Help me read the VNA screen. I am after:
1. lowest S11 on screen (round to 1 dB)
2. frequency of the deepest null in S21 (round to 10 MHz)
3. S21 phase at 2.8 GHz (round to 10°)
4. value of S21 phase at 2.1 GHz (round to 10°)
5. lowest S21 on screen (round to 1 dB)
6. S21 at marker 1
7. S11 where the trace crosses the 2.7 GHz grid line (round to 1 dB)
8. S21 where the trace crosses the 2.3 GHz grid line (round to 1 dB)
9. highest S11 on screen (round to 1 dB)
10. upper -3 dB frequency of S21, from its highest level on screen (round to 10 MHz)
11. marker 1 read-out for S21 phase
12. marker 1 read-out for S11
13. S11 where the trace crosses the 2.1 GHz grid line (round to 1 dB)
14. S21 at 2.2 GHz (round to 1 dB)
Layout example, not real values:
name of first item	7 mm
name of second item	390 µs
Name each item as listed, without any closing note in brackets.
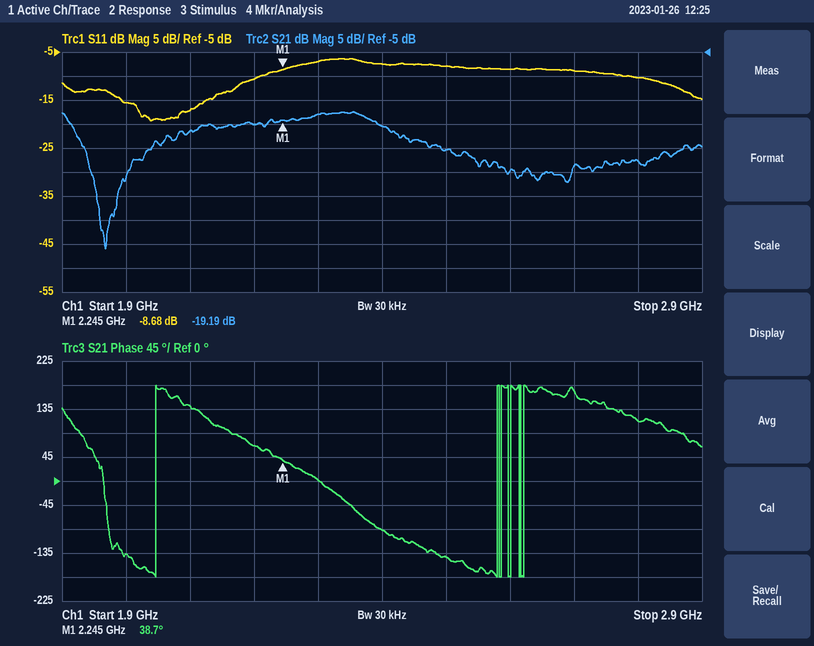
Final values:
lowest S11 on screen	-19 dB
frequency of the deepest null in S21	1.97 GHz
S21 phase at 2.8 GHz	110°
value of S21 phase at 2.1 GHz	140°
lowest S21 on screen	-46 dB
S21 at marker 1	-19.19 dB
S11 where the trace crosses the 2.7 GHz grid line	-9 dB
S21 where the trace crosses the 2.3 GHz grid line	-18 dB
highest S11 on screen	-6 dB
upper -3 dB frequency of S21, from its highest level on screen	2.40 GHz
marker 1 read-out for S21 phase	38.7°
marker 1 read-out for S11	-8.68 dB
S11 where the trace crosses the 2.1 GHz grid line	-17 dB
S21 at 2.2 GHz	-20 dB
